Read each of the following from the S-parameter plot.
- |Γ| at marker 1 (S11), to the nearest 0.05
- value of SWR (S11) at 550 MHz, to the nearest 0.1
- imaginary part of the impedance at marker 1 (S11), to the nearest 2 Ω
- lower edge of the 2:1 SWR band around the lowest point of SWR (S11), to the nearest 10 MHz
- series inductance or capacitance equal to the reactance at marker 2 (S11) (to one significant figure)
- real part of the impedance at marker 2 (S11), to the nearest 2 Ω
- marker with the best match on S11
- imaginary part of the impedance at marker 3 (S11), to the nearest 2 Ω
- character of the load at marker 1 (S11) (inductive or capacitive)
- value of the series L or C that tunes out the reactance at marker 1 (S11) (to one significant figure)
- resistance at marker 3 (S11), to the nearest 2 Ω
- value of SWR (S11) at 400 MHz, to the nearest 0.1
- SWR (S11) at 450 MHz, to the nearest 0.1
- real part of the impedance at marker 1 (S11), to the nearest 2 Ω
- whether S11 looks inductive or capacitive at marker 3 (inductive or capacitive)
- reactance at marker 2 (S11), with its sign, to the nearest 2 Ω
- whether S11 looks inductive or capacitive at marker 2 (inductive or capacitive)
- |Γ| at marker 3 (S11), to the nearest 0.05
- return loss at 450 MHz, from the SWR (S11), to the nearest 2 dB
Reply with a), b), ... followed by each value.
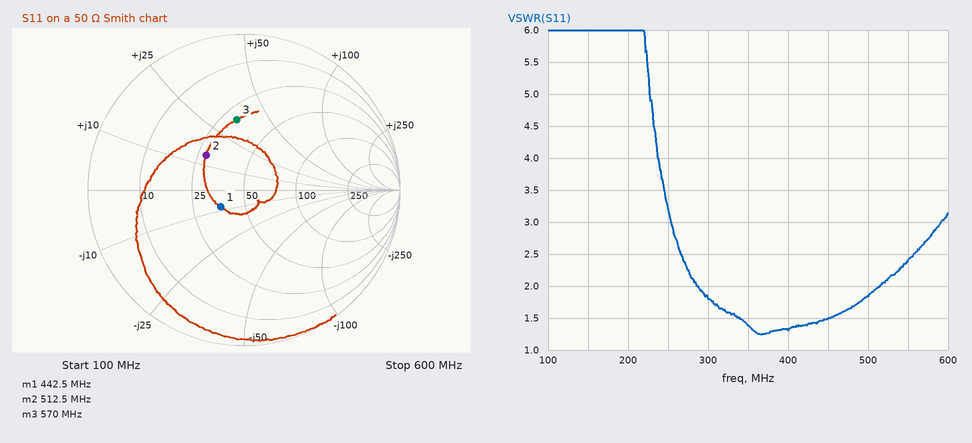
a) 0.20
b) 2.4
c) -8 Ω
d) 290 MHz
e) 4 nH
f) 28 Ω
g) marker 1
h) +34 Ω
i) capacitive
j) 3 nH
k) 30 Ω
l) 1.3
m) 1.5
n) 36 Ω
o) inductive
p) +14 Ω
q) inductive
r) 0.45
s) 14 dB
